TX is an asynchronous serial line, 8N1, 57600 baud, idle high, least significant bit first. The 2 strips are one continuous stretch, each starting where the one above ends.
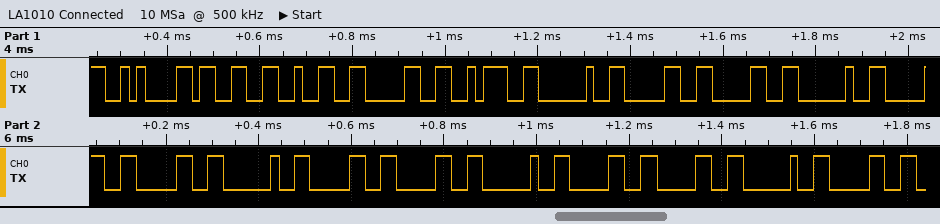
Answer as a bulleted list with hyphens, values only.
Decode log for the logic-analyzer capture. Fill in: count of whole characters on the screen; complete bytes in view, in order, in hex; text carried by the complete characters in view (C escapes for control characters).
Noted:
- 19
- 0A 33 32 30 3A 20 30 30 20 30 30 20 30 30 20 30 30 20 30
- "\n320: 00 00 00 00 0"
